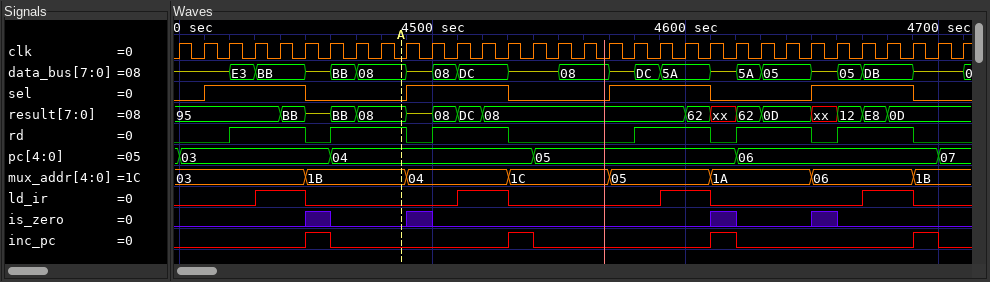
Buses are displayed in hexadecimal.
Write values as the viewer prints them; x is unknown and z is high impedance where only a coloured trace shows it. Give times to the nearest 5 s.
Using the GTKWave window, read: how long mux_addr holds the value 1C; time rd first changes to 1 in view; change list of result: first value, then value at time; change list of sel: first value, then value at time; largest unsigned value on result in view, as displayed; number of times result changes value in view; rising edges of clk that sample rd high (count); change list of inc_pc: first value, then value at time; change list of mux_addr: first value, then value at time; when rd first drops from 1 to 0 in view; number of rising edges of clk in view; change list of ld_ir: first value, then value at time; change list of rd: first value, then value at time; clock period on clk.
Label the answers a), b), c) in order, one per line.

a) 40 s
b) 4420 s
c) 95, BB at 4440 s, z at 4450 s, BB at 4460 s, 08 at 4470 s, z at 4490 s, 08 at 4500 s, DC at 4510 s, 08 at 4520 s, 62 at 4600 s, xx at 4610 s, 62 at 4620 s, 0D at 4630 s, xx at 4650 s, 12 at 4660 s, E8 at 4670 s, 0D at 4680 s
d) 0, 1 at 4410 s, 0 at 4450 s, 1 at 4490 s, 0 at 4530 s, 1 at 4570 s, 0 at 4610 s, 1 at 4650 s, 0 at 4690 s
e) E8
f) 16
g) 18
h) 0, 1 at 4450 s, 0 at 4460 s, 1 at 4530 s, 0 at 4540 s, 1 at 4610 s, 0 at 4620 s, 1 at 4690 s, 0 at 4700 s
i) 03, 1B at 4450 s, 04 at 4490 s, 1C at 4530 s, 05 at 4570 s, 1A at 4610 s, 06 at 4650 s, 1B at 4690 s
j) 4450 s
k) 32
l) 0, 1 at 4430 s, 0 at 4450 s, 1 at 4510 s, 0 at 4530 s, 1 at 4590 s, 0 at 4610 s, 1 at 4670 s, 0 at 4690 s
m) 0, 1 at 4420 s, 0 at 4450 s, 1 at 4460 s, 0 at 4490 s, 1 at 4500 s, 0 at 4530 s, 1 at 4580 s, 0 at 4610 s, 1 at 4620 s, 0 at 4650 s, 1 at 4660 s, 0 at 4690 s
n) 10 s
